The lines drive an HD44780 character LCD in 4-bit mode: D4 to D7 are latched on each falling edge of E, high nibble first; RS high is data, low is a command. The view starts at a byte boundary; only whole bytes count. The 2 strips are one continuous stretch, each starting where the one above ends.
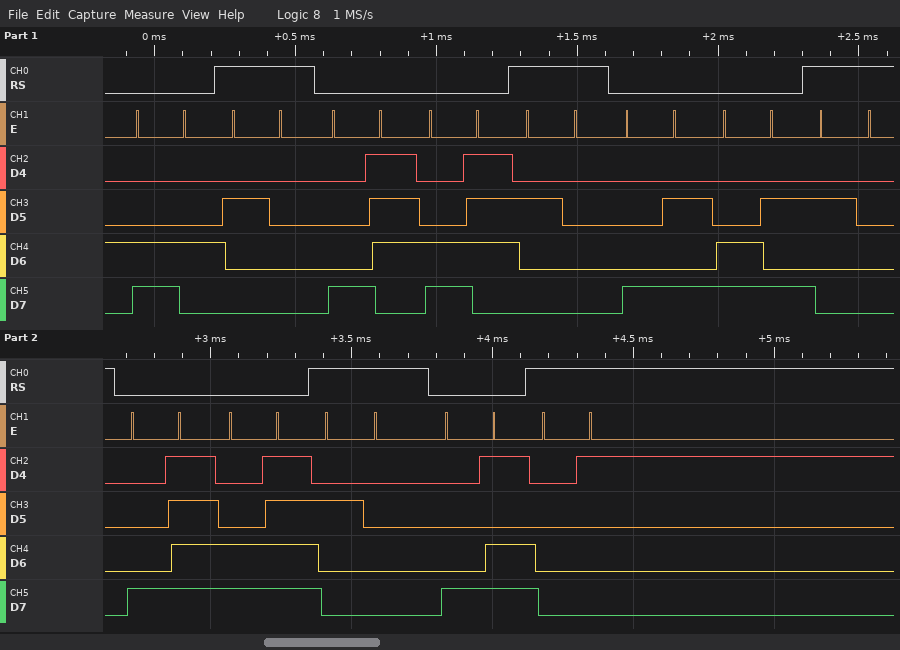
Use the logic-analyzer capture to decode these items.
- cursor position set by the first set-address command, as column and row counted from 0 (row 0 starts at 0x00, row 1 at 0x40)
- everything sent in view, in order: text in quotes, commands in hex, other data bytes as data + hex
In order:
column 4, row 1
0xC4 " " 0x87 0xC7 " " 0x8A 0xCA " " 0x8F 0xCF " " 0x8D data 01
